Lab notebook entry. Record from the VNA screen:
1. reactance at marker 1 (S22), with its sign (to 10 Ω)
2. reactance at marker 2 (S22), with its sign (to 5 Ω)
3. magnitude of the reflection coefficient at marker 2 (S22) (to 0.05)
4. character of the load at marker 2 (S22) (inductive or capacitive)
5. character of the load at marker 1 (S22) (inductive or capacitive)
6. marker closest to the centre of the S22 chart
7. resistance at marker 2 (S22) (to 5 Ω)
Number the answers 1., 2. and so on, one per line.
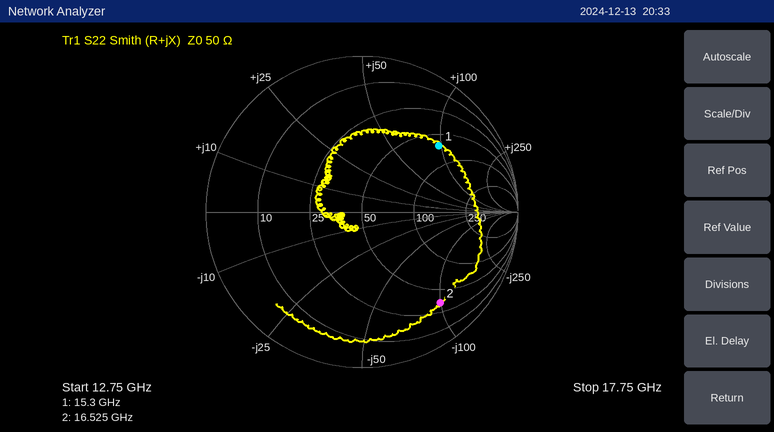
1. +100 Ω
2. -100 Ω
3. 0.75
4. capacitive
5. inductive
6. marker 1
7. 35 Ω
